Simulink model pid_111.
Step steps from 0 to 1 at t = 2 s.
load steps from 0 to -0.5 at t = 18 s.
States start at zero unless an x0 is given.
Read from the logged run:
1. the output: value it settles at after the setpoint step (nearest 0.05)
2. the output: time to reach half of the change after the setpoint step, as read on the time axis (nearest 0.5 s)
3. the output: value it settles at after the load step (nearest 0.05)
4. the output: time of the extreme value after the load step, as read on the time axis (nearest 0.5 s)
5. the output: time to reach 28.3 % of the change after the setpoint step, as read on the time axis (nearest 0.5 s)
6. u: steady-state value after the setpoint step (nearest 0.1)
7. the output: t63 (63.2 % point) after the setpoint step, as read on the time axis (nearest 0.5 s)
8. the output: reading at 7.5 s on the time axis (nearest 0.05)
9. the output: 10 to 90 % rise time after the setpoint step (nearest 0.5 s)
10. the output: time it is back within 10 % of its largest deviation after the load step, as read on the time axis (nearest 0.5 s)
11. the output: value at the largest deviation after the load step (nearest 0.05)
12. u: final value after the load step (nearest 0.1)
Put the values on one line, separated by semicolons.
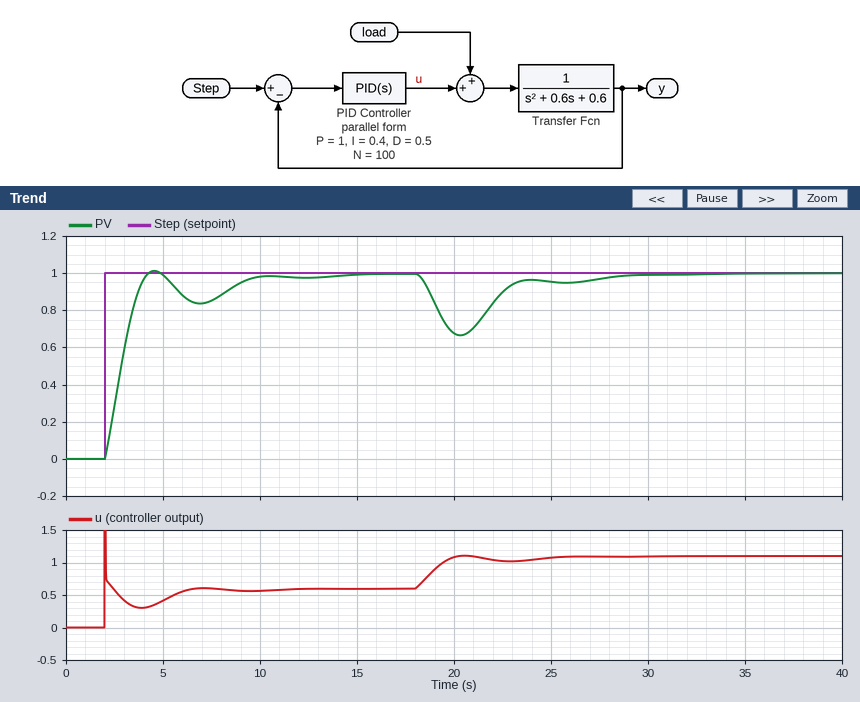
1.00; 3.0 s; 1.00; 20.5 s; 2.5 s; 0.6; 3.0 s; 0.85; 1.5 s; 27.5 s; 0.65; 1.1
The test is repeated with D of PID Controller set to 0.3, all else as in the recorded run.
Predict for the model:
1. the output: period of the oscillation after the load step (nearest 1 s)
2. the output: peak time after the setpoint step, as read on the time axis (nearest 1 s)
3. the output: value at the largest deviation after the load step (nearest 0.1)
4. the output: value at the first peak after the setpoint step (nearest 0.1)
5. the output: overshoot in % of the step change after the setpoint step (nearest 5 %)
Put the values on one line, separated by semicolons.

5 s; 5 s; 0.6; 1.1; 10 %
